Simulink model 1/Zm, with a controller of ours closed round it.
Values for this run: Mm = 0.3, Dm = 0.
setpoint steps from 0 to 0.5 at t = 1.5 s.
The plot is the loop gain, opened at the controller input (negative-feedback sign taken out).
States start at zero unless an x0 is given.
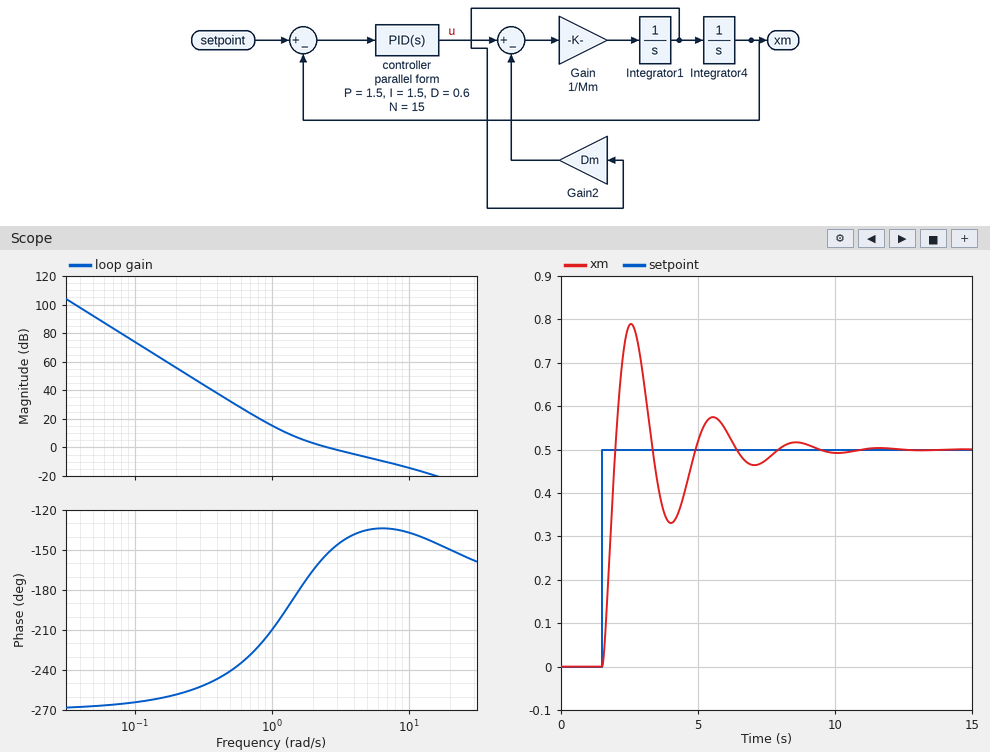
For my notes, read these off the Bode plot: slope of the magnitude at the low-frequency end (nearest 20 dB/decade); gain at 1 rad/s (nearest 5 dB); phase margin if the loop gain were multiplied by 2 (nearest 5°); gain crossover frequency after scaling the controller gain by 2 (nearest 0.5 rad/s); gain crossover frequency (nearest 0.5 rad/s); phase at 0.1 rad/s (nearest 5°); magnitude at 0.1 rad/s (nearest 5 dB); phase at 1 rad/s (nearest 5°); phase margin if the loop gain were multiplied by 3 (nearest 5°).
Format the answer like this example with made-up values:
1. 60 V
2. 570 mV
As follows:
1. -60 dB/decade
2. 15 dB
3. 45°
4. 4.5 rad/s
5. 2.5 rad/s
6. -265°
7. 75 dB
8. -210°
9. 45°
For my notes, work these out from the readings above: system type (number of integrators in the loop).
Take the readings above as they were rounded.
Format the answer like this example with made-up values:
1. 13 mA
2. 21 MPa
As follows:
1. 3
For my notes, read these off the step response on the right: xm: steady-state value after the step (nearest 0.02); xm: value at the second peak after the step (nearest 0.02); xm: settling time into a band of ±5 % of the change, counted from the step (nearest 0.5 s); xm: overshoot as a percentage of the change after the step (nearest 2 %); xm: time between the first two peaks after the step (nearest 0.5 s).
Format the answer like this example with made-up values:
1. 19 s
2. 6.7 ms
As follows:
1. 0.50
2. 0.58
3. 6.0 s
4. 58 %
5. 3.0 s
